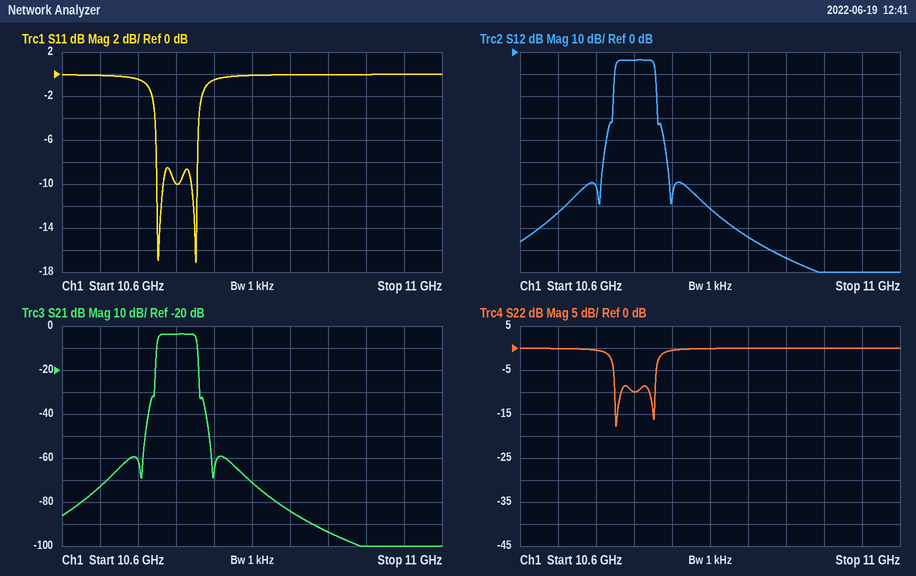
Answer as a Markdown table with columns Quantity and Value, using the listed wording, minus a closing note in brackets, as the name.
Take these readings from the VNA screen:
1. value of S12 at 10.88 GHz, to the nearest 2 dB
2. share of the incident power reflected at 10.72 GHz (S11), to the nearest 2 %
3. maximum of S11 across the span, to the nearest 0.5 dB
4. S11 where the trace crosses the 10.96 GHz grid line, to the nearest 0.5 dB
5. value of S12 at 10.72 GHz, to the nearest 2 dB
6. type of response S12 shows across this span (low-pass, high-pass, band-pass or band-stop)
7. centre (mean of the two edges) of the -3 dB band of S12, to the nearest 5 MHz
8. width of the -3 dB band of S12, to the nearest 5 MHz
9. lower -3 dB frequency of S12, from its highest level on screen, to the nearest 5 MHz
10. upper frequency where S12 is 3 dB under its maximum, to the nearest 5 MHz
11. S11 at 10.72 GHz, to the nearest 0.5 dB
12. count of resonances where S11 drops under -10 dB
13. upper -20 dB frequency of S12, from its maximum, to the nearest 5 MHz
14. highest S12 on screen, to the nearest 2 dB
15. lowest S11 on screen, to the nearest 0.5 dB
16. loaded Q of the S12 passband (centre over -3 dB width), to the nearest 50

| Quantity | Value |
|---|---|
| value of S12 at 10.88 GHz, to the nearest 2 dB | -94 dB |
| share of the incident power reflected at 10.72 GHz (S11), to the nearest 2 % | 10 % |
| maximum of S11 across the span, to the nearest 0.5 dB | 0.0 dB |
| S11 where the trace crosses the 10.96 GHz grid line, to the nearest 0.5 dB | 0.0 dB |
| value of S12 at 10.72 GHz, to the nearest 2 dB | -4 dB |
| type of response S12 shows across this span | band-pass |
| centre (mean of the two edges) of the -3 dB band of S12, to the nearest 5 MHz | 10.720 GHz |
| width of the -3 dB band of S12, to the nearest 5 MHz | 40 MHz |
| lower -3 dB frequency of S12, from its highest level on screen, to the nearest 5 MHz | 10.700 GHz |
| upper frequency where S12 is 3 dB under its maximum, to the nearest 5 MHz | 10.740 GHz |
| S11 at 10.72 GHz, to the nearest 0.5 dB | -10.0 dB |
| count of resonances where S11 drops under -10 dB | 2 |
| upper -20 dB frequency of S12, from its maximum, to the nearest 5 MHz | 10.745 GHz |
| highest S12 on screen, to the nearest 2 dB | -4 dB |
| lowest S11 on screen, to the nearest 0.5 dB | -17.0 dB |
| loaded Q of the S12 passband (centre over -3 dB width), to the nearest 50 | 250 |
